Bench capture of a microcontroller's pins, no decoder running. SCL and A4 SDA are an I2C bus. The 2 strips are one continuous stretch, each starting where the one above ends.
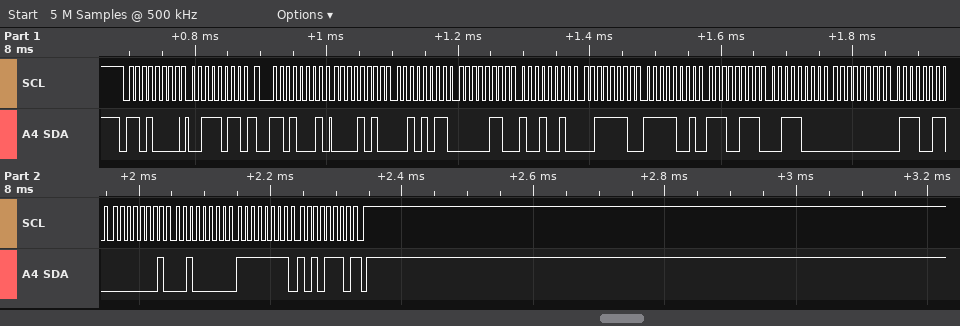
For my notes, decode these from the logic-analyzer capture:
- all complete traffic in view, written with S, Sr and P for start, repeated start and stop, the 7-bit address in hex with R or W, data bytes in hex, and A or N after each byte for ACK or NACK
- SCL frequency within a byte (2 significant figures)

S 68W A 3B A Sr 68R A 0A A 2B A 06 A 92 A 3E A F9 A E7 A 38 A 00 A 73 A 01 A 20 A FF A AE N P
100 kHz
